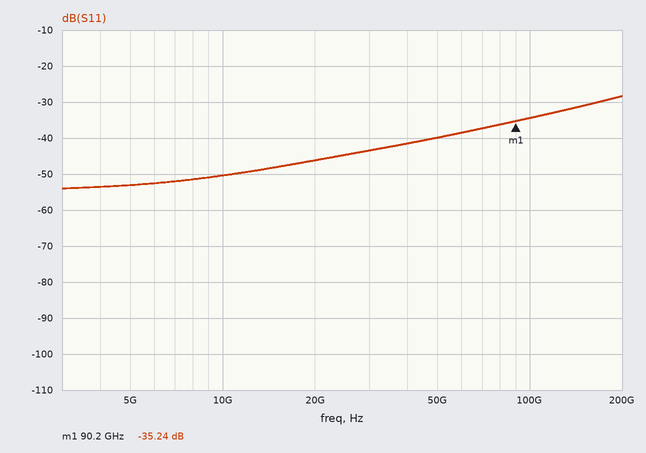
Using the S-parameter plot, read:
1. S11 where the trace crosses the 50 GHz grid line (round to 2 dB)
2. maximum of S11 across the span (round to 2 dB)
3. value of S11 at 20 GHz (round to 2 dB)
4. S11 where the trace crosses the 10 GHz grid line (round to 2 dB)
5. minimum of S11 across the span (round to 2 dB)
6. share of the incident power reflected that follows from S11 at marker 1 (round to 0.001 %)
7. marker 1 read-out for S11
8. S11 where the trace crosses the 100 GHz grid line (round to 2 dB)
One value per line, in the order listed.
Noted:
-40 dB
-28 dB
-46 dB
-50 dB
-54 dB
0.030 %
-35.24 dB
-34 dB
